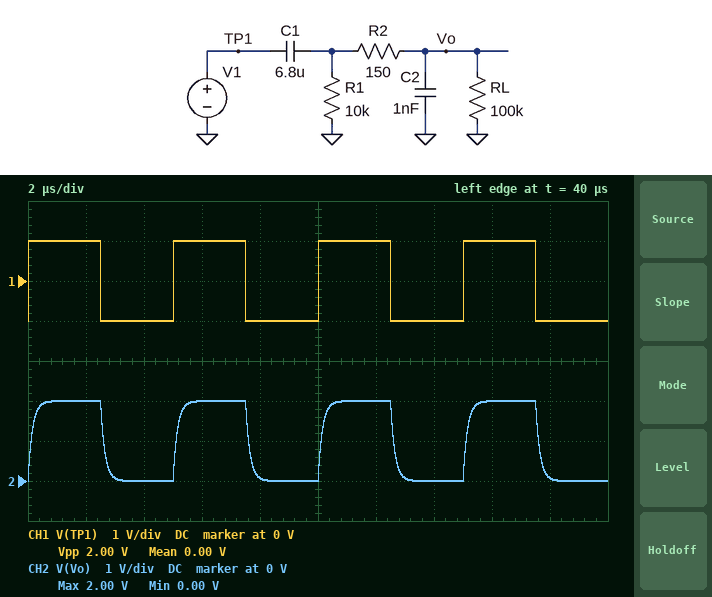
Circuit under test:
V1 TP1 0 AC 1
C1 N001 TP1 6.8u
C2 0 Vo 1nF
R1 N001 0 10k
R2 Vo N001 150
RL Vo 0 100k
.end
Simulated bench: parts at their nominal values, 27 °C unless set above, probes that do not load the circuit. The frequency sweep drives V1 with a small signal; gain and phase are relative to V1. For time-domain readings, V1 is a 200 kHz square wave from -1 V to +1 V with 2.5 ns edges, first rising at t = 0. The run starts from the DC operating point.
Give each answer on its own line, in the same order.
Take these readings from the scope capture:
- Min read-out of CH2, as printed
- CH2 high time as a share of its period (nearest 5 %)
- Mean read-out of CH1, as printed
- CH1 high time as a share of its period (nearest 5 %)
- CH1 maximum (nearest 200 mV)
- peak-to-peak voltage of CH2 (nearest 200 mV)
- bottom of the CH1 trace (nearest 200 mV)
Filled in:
0.00 V
50 %
0.00 V
50 %
1.0 V
2.0 V
-1.0 V
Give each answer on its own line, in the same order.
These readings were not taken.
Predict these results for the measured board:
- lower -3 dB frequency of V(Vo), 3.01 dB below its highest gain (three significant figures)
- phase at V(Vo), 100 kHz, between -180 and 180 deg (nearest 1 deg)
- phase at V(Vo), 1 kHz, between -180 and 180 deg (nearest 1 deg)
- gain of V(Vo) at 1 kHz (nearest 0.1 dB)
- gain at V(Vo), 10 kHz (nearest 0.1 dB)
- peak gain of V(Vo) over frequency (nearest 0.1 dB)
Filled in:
2.57 Hz
-5 deg
0 deg
0 dB
0 dB
0 dB
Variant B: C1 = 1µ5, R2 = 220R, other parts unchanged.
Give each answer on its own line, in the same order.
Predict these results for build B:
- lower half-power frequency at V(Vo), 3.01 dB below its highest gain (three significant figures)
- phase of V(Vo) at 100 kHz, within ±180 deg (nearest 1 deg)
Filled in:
11.7 Hz
-8 deg
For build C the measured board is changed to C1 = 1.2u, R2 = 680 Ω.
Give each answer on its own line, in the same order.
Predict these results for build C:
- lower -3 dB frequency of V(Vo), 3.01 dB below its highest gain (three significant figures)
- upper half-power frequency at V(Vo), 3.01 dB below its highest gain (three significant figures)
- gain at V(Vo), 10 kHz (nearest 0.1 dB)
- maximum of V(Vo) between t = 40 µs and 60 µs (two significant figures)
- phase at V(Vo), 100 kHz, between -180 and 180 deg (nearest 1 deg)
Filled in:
14.6 Hz
236 kHz
-0.1 dB
1.9 V
-23 deg
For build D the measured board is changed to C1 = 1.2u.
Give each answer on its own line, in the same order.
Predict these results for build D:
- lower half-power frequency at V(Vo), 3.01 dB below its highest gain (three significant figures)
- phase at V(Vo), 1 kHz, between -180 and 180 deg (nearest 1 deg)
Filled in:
14.6 Hz
1 deg
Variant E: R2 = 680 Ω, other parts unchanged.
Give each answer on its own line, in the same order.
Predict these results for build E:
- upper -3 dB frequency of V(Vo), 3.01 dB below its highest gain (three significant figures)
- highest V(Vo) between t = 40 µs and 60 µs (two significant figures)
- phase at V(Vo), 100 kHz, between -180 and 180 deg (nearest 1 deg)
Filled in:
236 kHz
1.9 V
-23 deg
